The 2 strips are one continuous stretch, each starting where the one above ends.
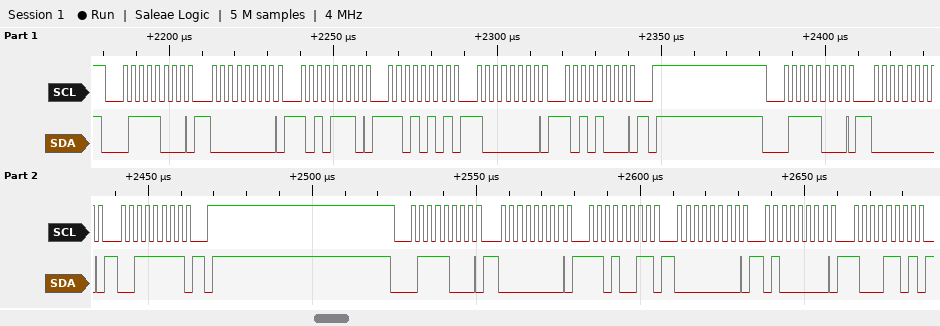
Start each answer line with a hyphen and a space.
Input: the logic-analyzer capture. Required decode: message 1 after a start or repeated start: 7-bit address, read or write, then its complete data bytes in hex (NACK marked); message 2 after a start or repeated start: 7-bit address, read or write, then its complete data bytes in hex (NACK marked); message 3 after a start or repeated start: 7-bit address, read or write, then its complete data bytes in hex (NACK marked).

- 0x3C write: 00 AE D5 80 A8
- 0x3C write: 00 3F
- 0x3C write: 00 D3 00 40 8D
